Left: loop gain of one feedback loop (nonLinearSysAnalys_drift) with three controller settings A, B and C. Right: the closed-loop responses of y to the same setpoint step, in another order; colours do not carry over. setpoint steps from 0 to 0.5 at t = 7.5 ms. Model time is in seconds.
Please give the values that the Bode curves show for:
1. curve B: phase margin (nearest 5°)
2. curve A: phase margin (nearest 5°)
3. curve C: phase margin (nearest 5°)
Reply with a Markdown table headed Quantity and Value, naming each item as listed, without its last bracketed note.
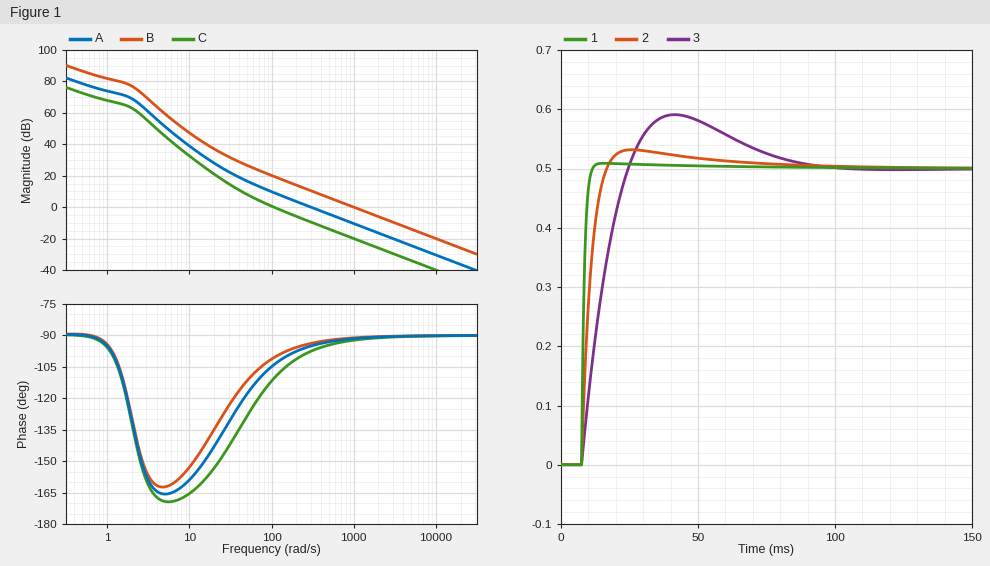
| Quantity | Value |
|---|---|
| curve B: phase margin | 90° |
| curve A: phase margin | 85° |
| curve C: phase margin | 70° |
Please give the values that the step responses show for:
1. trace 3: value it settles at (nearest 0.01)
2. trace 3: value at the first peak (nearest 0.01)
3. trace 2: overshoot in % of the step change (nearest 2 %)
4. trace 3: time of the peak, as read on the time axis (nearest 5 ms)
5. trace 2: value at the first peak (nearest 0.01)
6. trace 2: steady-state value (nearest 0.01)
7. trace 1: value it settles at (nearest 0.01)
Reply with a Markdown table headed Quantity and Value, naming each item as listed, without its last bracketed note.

| Quantity | Value |
|---|---|
| trace 3: value it settles at | 0.50 |
| trace 3: value at the first peak | 0.59 |
| trace 2: overshoot in % of the step change | 6 % |
| trace 3: time of the peak, as read on the time axis | 40 ms |
| trace 2: value at the first peak | 0.53 |
| trace 2: steady-state value | 0.50 |
| trace 1: value it settles at | 0.50 |
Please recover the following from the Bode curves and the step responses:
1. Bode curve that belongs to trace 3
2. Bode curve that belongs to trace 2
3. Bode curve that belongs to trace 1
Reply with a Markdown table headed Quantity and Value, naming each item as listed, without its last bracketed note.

| Quantity | Value |
|---|---|
| Bode curve that belongs to trace 3 | C |
| Bode curve that belongs to trace 2 | A |
| Bode curve that belongs to trace 1 | B |
